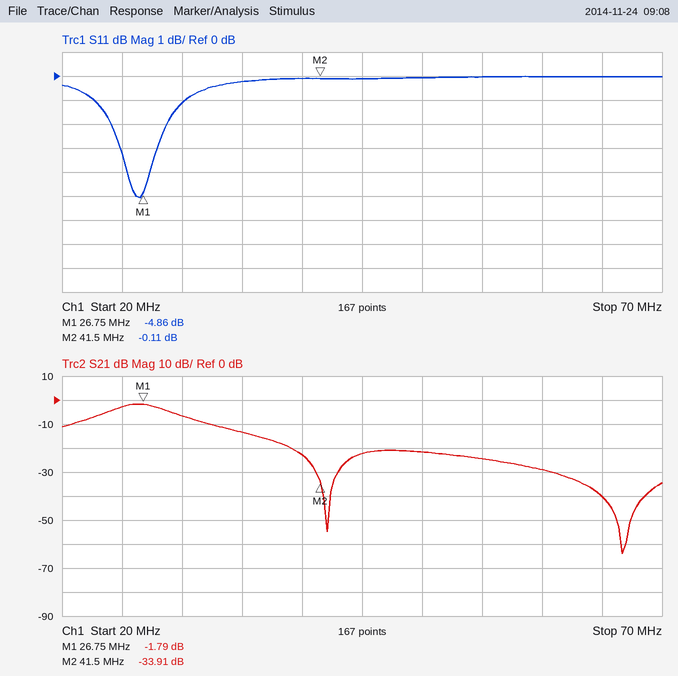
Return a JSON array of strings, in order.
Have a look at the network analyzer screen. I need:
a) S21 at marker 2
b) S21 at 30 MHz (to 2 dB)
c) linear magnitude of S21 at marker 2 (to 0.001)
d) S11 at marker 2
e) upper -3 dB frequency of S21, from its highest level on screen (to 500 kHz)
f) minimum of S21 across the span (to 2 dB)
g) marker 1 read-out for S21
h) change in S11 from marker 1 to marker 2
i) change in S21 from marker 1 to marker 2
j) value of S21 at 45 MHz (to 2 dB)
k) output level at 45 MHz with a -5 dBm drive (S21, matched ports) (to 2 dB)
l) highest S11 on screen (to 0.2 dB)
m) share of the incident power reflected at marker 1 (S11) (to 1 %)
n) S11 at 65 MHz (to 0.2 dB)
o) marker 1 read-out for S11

["-33.91 dB", "-6 dB", "0.020", "-0.11 dB", "29.0 MHz", "-64 dB", "-1.79 dB", "4.75 dB", "-32.12 dB", "-22 dB", "-28 dBm", "0.0 dB", "33 %", "0.0 dB", "-4.86 dB"]
